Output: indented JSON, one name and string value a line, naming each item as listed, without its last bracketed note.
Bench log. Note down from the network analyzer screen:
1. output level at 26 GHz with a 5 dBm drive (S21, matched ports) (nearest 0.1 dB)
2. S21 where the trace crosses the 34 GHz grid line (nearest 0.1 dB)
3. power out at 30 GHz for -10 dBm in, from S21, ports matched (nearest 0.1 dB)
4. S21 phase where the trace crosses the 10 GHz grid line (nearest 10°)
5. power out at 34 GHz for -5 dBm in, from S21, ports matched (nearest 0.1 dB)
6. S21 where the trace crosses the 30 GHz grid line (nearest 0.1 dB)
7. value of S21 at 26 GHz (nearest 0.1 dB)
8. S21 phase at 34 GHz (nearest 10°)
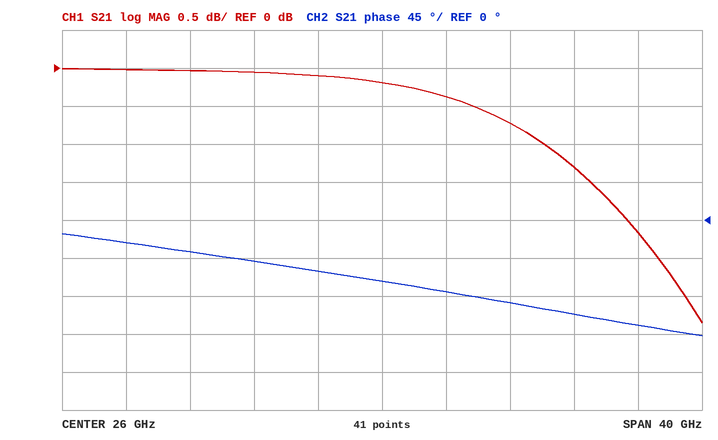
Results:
{
  "output level at 26 GHz with a 5 dBm drive (S21, matched ports)": "4.8 dBm",
  "S21 where the trace crosses the 34 GHz grid line": "-0.7 dB",
  "power out at 30 GHz for -10 dBm in, from S21, ports matched": "-10.4 dBm",
  "S21 phase where the trace crosses the 10 GHz grid line": "-30°",
  "power out at 34 GHz for -5 dBm in, from S21, ports matched": "-5.7 dBm",
  "S21 where the trace crosses the 30 GHz grid line": "-0.4 dB",
  "value of S21 at 26 GHz": "-0.2 dB",
  "S21 phase at 34 GHz": "-100°"
}
